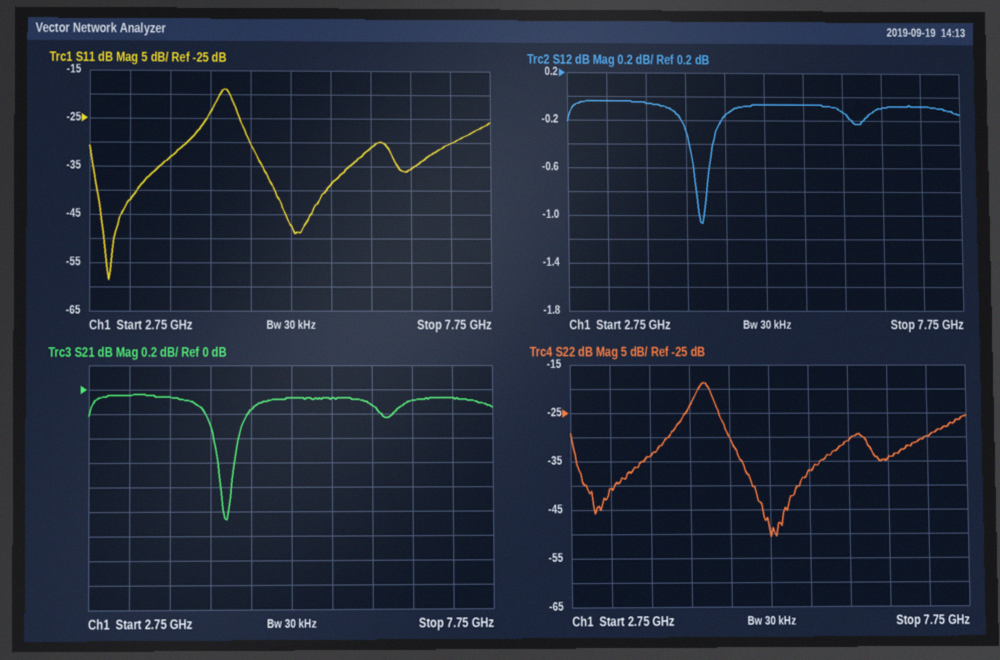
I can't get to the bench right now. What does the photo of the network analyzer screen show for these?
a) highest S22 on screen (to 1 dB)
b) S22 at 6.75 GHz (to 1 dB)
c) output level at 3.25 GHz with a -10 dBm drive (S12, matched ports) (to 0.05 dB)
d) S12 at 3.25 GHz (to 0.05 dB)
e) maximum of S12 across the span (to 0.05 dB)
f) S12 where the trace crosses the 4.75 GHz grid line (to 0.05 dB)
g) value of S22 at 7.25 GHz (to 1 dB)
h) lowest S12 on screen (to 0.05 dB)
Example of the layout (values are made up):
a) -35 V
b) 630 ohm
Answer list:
a) -19 dB
b) -34 dB
c) -10.05 dBm
d) -0.05 dB
e) -0.05 dB
f) -0.15 dB
g) -30 dB
h) -1.05 dB
